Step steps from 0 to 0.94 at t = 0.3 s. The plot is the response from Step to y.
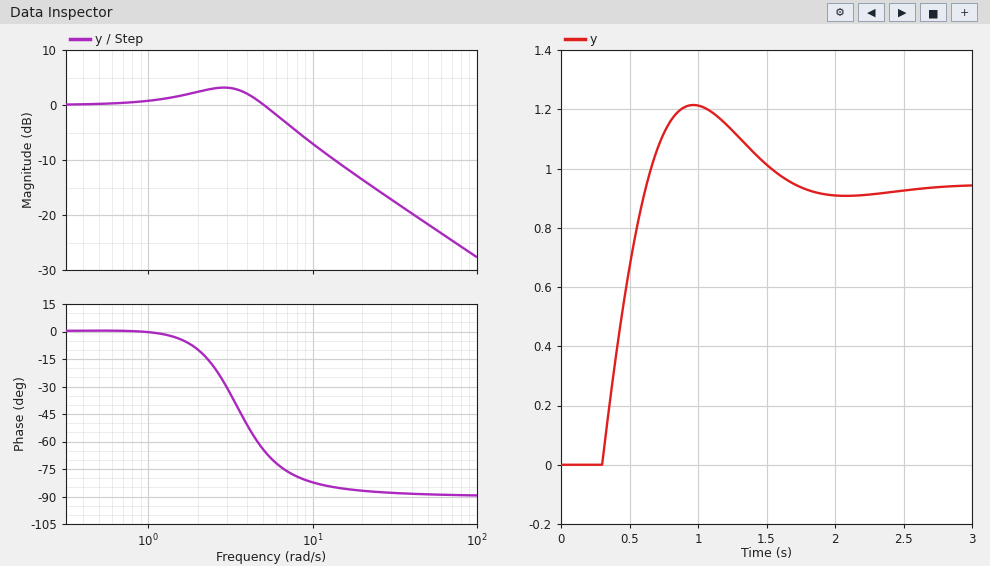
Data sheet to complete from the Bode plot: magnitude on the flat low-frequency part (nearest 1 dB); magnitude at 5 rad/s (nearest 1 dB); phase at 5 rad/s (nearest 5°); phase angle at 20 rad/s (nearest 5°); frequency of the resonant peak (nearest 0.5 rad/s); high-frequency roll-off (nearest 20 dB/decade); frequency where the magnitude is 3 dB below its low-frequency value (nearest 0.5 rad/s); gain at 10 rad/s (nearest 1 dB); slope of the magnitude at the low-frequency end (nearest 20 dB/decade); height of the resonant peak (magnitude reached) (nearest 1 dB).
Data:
0 dB
0 dB
-65°
-85°
3.0 rad/s
-20 dB/decade
6.5 rad/s
-7 dB
0 dB/decade
3 dB
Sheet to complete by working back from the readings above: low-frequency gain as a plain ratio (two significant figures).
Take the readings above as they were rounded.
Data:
1.0
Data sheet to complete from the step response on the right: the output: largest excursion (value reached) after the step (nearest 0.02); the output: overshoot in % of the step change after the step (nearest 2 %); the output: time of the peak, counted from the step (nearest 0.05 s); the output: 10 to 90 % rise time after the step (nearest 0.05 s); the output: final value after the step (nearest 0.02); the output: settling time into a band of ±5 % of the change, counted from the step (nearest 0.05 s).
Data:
1.22
30 %
0.65 s
0.25 s
0.94
1.25 s
